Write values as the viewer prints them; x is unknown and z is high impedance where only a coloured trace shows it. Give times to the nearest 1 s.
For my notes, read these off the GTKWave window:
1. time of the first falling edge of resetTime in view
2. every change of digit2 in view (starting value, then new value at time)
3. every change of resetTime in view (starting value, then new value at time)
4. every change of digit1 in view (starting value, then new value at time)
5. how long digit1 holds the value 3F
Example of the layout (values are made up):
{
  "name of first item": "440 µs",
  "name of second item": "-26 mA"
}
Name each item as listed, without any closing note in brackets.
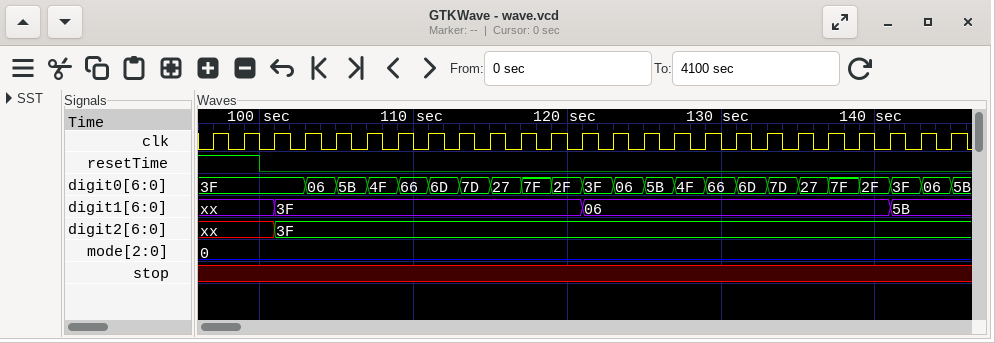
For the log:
{
  "time of the first falling edge of resetTime in view": "100 s",
  "every change of digit2 in view": "xx, 3F at 101 s",
  "every change of resetTime in view": "1, 0 at 100 s",
  "every change of digit1 in view": "xx, 3F at 101 s, 06 at 121 s, 5B at 141 s",
  "how long digit1 holds the value 3F": "20 s"
}
